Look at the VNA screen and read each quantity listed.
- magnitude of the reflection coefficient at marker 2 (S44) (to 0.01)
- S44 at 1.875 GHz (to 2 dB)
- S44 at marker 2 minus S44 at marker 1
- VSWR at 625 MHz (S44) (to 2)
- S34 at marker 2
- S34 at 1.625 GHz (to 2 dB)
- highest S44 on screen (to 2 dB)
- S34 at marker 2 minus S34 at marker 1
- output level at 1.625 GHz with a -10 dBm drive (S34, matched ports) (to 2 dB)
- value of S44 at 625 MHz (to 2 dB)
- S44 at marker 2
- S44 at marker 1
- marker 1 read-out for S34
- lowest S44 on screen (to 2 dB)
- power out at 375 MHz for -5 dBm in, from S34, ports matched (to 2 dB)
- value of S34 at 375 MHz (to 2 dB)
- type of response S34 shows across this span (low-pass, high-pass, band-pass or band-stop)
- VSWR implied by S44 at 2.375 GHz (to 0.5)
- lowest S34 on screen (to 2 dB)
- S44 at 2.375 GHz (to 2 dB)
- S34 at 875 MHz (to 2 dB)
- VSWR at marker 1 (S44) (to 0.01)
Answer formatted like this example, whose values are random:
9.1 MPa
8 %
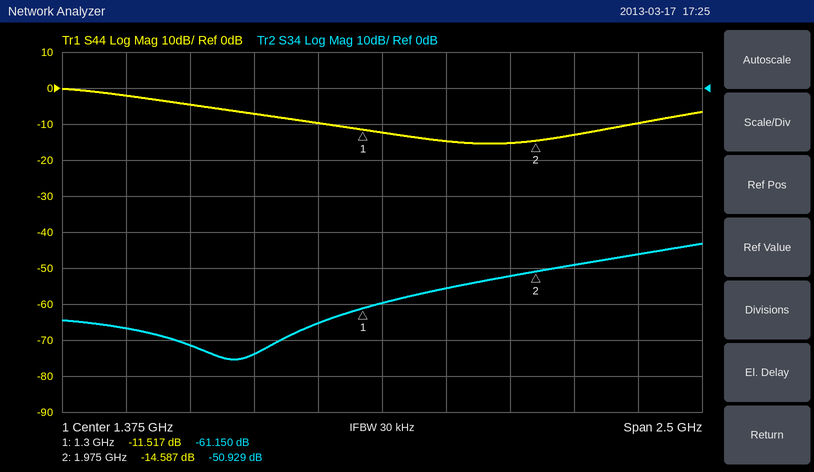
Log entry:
0.19
-16 dB
-3.070 dB
4
-50.929 dB
-56 dB
0 dB
10.221 dB
-66 dBm
-4 dB
-14.587 dB
-11.517 dB
-61.150 dB
-16 dB
-72 dBm
-66 dB
high-pass
2.0
-76 dB
-10 dB
-74 dB
1.72
